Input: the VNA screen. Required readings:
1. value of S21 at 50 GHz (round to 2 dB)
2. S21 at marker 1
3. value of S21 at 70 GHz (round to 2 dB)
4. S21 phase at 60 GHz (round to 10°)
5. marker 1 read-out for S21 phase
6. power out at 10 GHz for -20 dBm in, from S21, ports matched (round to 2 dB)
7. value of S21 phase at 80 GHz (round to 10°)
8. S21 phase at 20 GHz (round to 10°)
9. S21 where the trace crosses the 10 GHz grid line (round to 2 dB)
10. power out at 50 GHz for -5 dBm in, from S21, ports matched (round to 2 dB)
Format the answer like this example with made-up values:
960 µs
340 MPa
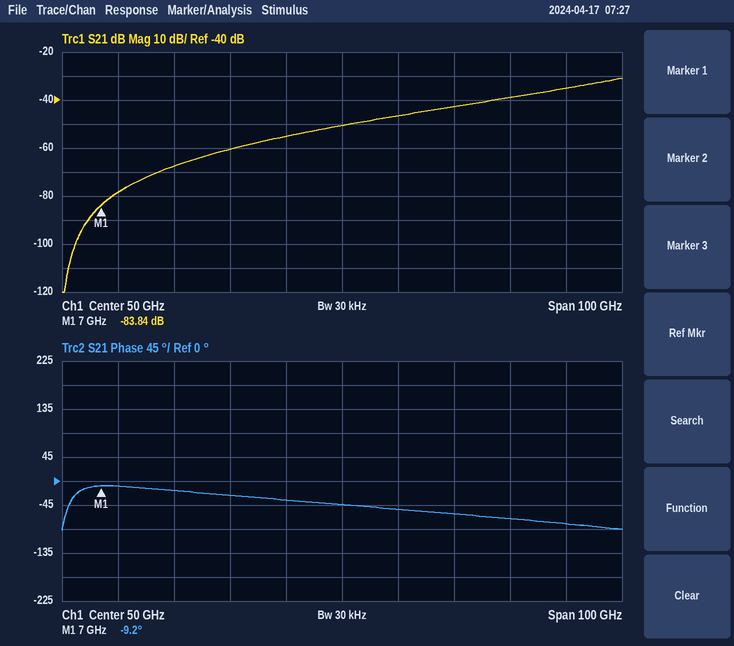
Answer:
-50 dB
-83.84 dB
-42 dB
-50°
-9.2°
-98 dBm
-70°
-20°
-78 dB
-56 dBm
